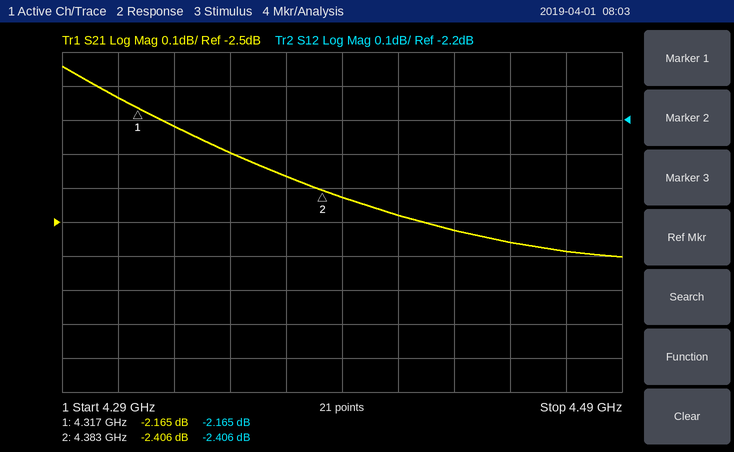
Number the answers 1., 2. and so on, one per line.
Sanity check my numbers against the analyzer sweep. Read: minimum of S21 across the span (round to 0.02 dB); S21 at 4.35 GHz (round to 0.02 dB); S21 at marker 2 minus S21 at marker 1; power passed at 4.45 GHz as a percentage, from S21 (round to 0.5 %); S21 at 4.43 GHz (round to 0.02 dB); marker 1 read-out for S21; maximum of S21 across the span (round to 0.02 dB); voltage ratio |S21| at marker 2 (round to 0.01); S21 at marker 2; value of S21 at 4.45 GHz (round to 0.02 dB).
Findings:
1. -2.60 dB
2. -2.30 dB
3. -0.241 dB
4. 55.5 %
5. -2.52 dB
6. -2.165 dB
7. -2.04 dB
8. 0.76
9. -2.406 dB
10. -2.56 dB
